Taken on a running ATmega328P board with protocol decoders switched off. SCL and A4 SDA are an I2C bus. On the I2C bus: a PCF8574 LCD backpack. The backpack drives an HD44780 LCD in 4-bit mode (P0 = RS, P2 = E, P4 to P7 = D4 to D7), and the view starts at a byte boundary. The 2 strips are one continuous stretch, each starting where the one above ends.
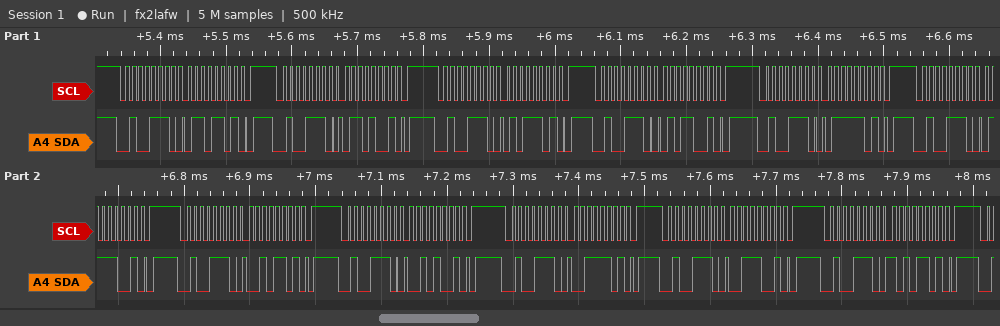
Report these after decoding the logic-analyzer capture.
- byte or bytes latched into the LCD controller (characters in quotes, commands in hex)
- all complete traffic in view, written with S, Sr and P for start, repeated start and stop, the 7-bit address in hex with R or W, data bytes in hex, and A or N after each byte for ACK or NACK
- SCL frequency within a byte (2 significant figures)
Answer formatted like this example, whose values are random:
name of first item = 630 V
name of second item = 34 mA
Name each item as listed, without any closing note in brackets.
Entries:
byte or bytes latched into the LCD controller = 'e' 'r'
all complete traffic in view, written with S, Sr and P for start, repeated start and stop, the 7-bit address in hex with R or W, data bytes in hex, and A or N after each byte for ACK or NACK = S 27W A 6D A P S 27W A 69 A P S 27W A 5D A P S 27W A 59 A P S 27W A 7D A P S 27W A 79 A P S 27W A 2D A P S 27W A 29 A P S 27W A 3D A P S 27W A 39 A P S 27W A AD A P
SCL frequency within a byte = 100 kHz
